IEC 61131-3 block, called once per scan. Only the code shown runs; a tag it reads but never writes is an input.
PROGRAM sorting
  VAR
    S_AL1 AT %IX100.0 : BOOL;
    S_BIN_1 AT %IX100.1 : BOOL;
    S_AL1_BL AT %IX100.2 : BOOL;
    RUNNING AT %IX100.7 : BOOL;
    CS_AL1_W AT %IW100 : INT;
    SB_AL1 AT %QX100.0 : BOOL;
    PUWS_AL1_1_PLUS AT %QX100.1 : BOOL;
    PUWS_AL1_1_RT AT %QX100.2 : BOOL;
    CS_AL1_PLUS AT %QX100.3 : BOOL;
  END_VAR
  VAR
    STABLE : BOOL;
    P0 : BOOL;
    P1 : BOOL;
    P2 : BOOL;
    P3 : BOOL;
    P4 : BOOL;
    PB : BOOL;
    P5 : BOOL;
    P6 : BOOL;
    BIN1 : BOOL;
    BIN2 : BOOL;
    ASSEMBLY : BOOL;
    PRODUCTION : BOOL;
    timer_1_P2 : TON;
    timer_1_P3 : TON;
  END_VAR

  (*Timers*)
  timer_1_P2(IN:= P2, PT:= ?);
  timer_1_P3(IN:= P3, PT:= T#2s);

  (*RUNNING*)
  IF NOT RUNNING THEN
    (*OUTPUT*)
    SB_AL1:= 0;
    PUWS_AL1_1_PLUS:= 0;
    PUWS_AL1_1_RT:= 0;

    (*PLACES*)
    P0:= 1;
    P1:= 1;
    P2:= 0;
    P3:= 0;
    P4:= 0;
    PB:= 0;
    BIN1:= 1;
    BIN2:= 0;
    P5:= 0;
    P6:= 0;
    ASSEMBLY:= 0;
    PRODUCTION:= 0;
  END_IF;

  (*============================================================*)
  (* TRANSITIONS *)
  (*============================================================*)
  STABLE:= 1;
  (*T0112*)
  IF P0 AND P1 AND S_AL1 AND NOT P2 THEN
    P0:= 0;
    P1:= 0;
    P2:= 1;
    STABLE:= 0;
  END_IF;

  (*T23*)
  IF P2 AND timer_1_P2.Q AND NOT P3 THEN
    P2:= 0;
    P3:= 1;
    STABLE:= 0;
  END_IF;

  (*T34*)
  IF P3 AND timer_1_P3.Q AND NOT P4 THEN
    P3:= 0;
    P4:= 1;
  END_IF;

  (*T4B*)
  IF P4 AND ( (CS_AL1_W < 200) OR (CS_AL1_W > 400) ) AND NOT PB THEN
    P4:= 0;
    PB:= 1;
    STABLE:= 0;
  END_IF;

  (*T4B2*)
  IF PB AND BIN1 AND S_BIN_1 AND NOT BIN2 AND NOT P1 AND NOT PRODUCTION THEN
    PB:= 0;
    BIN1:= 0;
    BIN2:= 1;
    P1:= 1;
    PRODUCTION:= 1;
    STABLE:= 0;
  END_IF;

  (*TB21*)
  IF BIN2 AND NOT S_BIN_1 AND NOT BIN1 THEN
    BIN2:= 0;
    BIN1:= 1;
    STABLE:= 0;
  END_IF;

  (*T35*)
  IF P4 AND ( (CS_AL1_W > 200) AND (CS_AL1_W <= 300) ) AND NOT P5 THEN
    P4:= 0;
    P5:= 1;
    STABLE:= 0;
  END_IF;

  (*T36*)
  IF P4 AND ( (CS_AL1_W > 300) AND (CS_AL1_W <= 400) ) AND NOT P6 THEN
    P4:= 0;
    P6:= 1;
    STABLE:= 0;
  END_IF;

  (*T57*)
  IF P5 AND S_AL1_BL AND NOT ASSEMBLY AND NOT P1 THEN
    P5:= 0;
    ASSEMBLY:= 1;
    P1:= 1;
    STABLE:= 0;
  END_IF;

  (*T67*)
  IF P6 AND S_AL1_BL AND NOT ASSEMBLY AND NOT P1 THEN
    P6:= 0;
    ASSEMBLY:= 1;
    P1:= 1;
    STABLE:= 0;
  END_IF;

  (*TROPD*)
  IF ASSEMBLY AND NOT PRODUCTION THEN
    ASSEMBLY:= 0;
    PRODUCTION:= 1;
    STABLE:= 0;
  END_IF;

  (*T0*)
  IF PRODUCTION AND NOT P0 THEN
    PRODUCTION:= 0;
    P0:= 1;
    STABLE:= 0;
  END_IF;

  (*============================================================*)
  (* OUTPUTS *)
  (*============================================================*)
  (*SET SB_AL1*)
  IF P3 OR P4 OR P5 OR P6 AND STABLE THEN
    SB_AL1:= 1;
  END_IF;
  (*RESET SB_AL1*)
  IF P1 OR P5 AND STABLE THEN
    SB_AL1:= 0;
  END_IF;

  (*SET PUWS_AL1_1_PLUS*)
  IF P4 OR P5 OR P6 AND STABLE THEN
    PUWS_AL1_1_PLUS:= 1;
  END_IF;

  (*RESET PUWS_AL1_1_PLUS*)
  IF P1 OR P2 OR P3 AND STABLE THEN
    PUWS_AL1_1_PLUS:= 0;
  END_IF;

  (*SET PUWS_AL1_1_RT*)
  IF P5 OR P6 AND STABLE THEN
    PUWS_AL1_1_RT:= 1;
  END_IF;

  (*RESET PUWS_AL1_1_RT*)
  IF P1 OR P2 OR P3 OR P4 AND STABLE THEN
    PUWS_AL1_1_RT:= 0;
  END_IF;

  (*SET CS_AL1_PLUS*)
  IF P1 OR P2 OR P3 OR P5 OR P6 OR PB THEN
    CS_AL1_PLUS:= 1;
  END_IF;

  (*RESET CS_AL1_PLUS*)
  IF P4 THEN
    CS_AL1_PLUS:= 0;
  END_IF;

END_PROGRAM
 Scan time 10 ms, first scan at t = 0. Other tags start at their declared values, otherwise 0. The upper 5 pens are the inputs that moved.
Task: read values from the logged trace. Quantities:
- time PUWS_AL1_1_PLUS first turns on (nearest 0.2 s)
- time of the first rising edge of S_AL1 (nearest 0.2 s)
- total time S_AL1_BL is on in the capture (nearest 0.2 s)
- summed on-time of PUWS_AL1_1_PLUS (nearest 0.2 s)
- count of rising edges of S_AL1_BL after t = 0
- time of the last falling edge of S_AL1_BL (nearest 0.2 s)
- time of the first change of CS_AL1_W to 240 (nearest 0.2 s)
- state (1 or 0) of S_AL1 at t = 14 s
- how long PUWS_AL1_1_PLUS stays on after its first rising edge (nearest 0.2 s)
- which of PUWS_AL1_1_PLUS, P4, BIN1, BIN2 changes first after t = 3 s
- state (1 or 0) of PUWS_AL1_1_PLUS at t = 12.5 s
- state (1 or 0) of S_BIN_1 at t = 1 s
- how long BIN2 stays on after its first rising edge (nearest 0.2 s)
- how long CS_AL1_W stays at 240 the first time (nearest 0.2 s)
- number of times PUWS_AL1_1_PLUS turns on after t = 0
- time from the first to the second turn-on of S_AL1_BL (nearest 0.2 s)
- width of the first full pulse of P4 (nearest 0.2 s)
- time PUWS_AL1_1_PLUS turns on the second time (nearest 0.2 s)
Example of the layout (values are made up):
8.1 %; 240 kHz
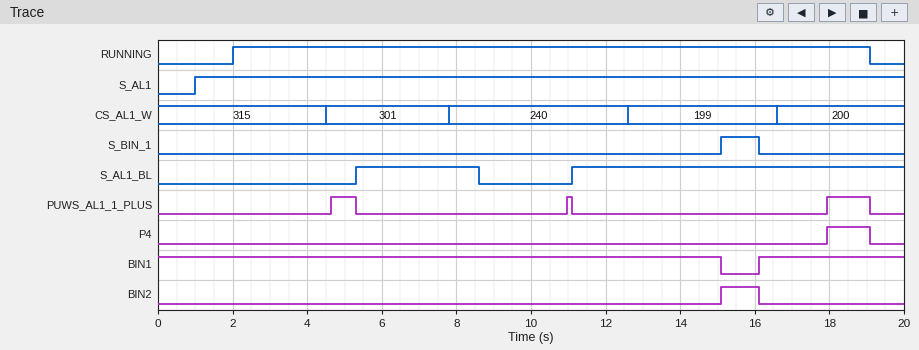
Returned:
4.6 s; 1.0 s; 12.2 s; 2.0 s; 2; 8.6 s; 7.8 s; 1; 0.6 s; PUWS_AL1_1_PLUS; 0; 0; 1.0 s; 4.8 s; 3; 5.8 s; 1.2 s; 11.0 s
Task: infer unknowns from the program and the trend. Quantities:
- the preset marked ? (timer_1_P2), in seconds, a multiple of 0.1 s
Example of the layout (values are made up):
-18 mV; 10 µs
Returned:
0.8 s
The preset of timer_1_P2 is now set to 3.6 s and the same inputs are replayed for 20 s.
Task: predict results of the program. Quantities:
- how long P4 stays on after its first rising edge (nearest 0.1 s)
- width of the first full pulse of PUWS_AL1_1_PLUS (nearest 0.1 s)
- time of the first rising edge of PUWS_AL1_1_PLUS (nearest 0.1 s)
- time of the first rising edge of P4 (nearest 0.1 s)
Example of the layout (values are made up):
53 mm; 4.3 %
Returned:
1.2 s; 1.2 s; 17.9 s; 17.9 s
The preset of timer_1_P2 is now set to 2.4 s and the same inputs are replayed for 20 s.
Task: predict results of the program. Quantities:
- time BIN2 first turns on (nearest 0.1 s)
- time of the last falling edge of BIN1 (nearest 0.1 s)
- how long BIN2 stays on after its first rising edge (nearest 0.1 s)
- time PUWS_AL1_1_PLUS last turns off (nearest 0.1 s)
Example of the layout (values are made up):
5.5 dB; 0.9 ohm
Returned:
15.5 s; 15.5 s; 0.6 s; 11.1 s
